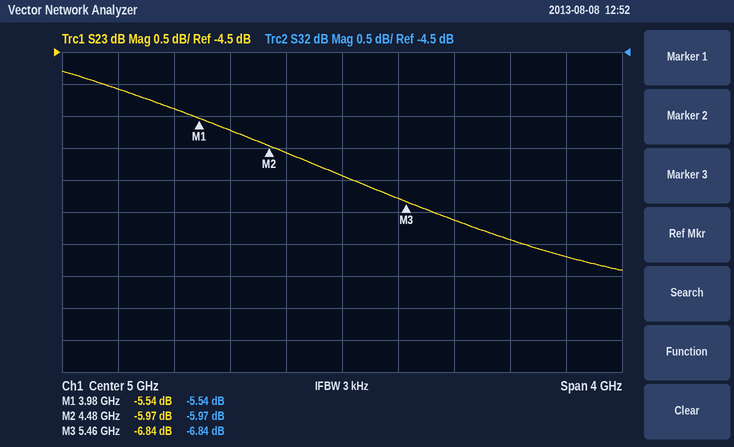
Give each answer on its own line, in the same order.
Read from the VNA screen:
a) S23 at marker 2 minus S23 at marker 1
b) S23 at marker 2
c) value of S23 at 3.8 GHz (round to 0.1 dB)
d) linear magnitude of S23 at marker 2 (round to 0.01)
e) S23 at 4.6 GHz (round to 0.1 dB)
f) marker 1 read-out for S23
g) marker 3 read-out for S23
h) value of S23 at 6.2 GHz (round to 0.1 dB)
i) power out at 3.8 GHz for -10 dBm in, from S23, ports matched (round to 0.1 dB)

-0.43 dB
-5.97 dB
-5.4 dB
0.50
-6.1 dB
-5.54 dB
-6.84 dB
-7.4 dB
-15.4 dBm
